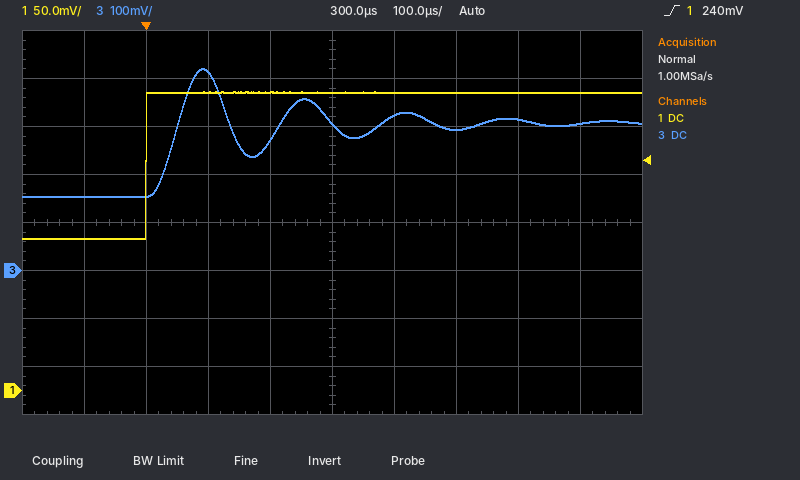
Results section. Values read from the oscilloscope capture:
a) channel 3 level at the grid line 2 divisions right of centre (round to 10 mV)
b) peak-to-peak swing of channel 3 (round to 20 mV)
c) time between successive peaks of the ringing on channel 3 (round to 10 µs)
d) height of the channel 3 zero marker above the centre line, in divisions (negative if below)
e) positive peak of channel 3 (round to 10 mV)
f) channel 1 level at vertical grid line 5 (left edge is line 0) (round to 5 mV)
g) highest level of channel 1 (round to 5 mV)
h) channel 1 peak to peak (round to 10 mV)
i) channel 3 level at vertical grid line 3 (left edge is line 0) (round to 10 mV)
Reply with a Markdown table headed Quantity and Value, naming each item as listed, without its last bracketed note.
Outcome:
| Quantity | Value |
|---|---|
| channel 3 level at the grid line 2 divisions right of centre | 290 mV |
| peak-to-peak swing of channel 3 | 260 mV |
| time between successive peaks of the ringing on channel 3 | 160 µs |
| height of the channel 3 zero marker above the centre line, in divisions | -1.0 div |
| positive peak of channel 3 | 420 mV |
| channel 1 level at vertical grid line 5 (left edge is line 0) | 310 mV |
| highest level of channel 1 | 310 mV |
| channel 1 peak to peak | 150 mV |
| channel 3 level at vertical grid line 3 (left edge is line 0) | 410 mV |
